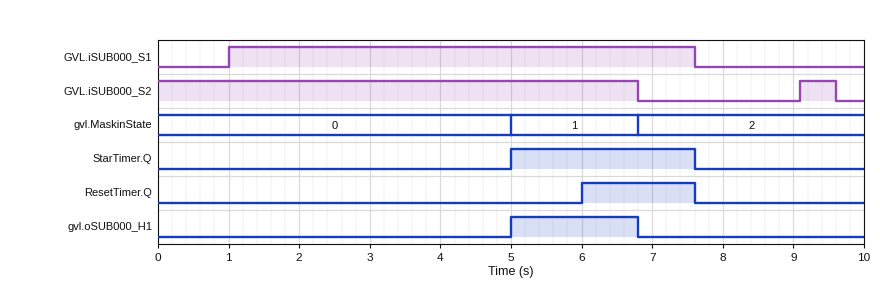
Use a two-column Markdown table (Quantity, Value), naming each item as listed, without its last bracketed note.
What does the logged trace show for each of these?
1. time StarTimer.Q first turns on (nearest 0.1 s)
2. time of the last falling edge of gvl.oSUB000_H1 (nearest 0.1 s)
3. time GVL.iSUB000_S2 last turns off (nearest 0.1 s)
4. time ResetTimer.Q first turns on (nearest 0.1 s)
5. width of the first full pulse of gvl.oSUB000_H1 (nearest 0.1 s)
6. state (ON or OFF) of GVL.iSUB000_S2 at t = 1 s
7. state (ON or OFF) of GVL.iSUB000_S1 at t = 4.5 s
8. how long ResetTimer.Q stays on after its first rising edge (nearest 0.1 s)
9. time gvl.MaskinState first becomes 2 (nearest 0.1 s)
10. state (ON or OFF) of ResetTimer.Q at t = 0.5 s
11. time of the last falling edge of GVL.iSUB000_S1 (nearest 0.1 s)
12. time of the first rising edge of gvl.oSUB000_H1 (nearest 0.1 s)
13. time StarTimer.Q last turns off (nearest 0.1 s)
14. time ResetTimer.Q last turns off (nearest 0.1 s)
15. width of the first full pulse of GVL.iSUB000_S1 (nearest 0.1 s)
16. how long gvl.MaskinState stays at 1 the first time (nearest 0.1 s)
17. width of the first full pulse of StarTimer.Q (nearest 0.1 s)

| Quantity | Value |
|---|---|
| time StarTimer.Q first turns on | 5.0 s |
| time of the last falling edge of gvl.oSUB000_H1 | 6.8 s |
| time GVL.iSUB000_S2 last turns off | 9.6 s |
| time ResetTimer.Q first turns on | 6.0 s |
| width of the first full pulse of gvl.oSUB000_H1 | 1.8 s |
| state (ON or OFF) of GVL.iSUB000_S2 at t = 1 s | ON |
| state (ON or OFF) of GVL.iSUB000_S1 at t = 4.5 s | ON |
| how long ResetTimer.Q stays on after its first rising edge | 1.6 s |
| time gvl.MaskinState first becomes 2 | 6.8 s |
| state (ON or OFF) of ResetTimer.Q at t = 0.5 s | OFF |
| time of the last falling edge of GVL.iSUB000_S1 | 7.6 s |
| time of the first rising edge of gvl.oSUB000_H1 | 5.0 s |
| time StarTimer.Q last turns off | 7.6 s |
| time ResetTimer.Q last turns off | 7.6 s |
| width of the first full pulse of GVL.iSUB000_S1 | 6.6 s |
| how long gvl.MaskinState stays at 1 the first time | 1.8 s |
| width of the first full pulse of StarTimer.Q | 2.6 s |
